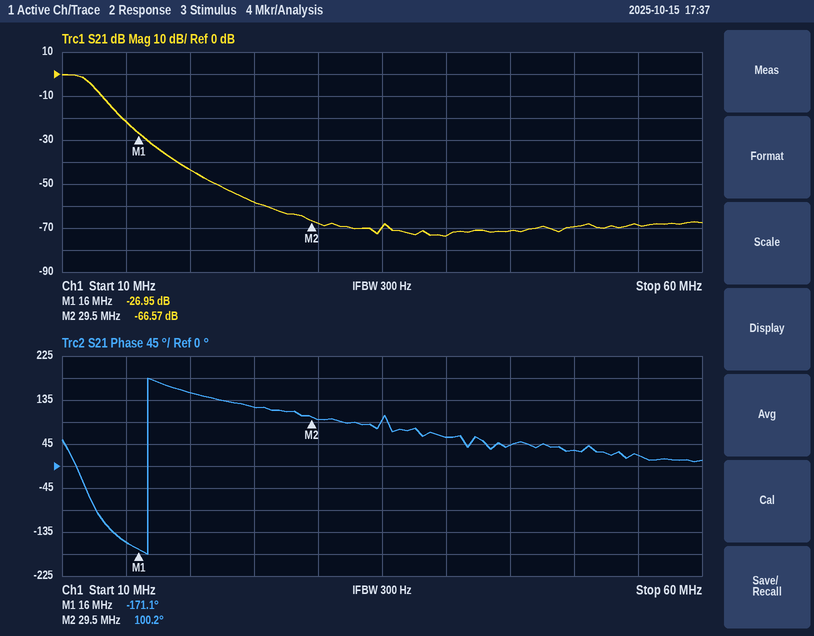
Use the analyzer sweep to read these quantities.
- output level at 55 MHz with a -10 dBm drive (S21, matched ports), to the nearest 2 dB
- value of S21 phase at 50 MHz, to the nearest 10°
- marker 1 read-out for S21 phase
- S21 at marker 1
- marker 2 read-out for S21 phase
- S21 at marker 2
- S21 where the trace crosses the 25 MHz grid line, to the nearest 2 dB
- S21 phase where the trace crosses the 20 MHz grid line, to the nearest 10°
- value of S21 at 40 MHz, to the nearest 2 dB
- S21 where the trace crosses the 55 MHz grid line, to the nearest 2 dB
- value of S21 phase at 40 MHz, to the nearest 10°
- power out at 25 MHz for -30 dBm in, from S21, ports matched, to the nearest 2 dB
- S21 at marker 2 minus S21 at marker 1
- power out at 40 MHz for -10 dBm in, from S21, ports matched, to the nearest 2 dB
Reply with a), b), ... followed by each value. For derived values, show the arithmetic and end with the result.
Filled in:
a) -10 dBm + (-68 dB) = -78 dBm
b) 30°
c) -171.1°
d) -26.95 dB
e) 100.2°
f) -66.57 dB
g) -58 dB
h) 150°
i) -74 dB
j) -68 dB
k) 60°
l) -30 dBm + (-58 dB) = -88 dBm
m) -66.57 − (-26.95) = -39.62 dB
n) -10 dBm + (-74 dB) = -84 dBm
